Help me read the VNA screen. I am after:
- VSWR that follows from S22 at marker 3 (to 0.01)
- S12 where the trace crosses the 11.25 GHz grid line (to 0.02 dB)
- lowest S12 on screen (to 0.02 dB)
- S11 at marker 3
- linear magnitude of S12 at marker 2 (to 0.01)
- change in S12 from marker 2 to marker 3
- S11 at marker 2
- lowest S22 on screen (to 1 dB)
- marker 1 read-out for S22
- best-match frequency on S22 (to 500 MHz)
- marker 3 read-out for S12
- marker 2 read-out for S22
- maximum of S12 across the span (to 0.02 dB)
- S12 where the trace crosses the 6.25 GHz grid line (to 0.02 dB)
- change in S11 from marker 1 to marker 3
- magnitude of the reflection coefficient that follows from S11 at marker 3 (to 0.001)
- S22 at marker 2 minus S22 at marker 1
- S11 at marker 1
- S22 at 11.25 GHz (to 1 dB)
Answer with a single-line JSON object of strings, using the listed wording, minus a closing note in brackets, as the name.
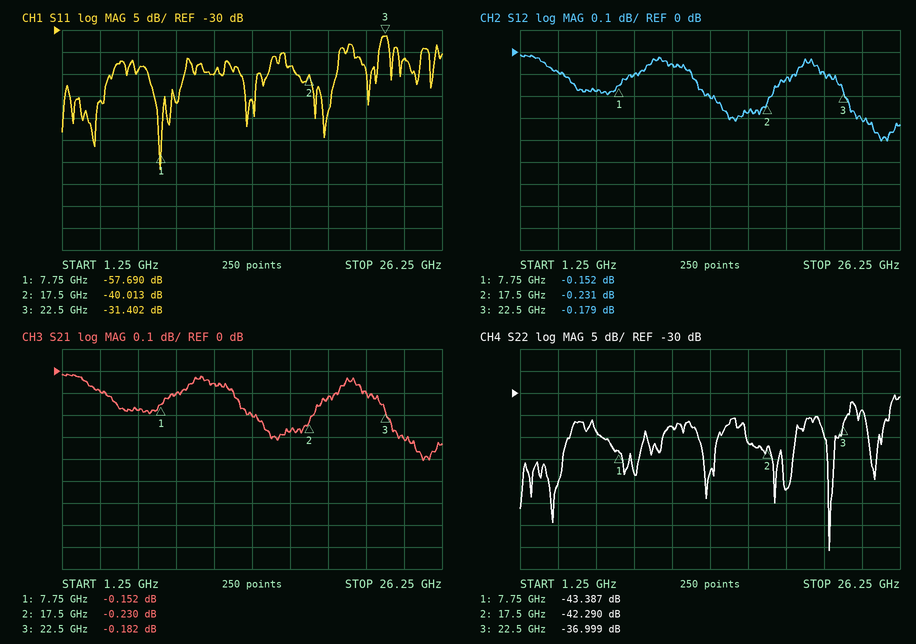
{"VSWR that follows from S22 at marker 3": "1.03", "S12 where the trace crosses the 11.25 GHz grid line": "-0.06 dB", "lowest S12 on screen": "-0.40 dB", "S11 at marker 3": "-31.402 dB", "linear magnitude of S12 at marker 2": "0.97", "change in S12 from marker 2 to marker 3": "0.052 dB", "S11 at marker 2": "-40.013 dB", "lowest S22 on screen": "-66 dB", "marker 1 read-out for S22": "-43.387 dB", "best-match frequency on S22": "21.5 GHz", "marker 3 read-out for S12": "-0.179 dB", "marker 2 read-out for S22": "-42.290 dB", "maximum of S12 across the span": "-0.02 dB", "S12 where the trace crosses the 6.25 GHz grid line": "-0.18 dB", "change in S11 from marker 1 to marker 3": "26.288 dB", "magnitude of the reflection coefficient that follows from S11 at marker 3": "0.027", "S22 at marker 2 minus S22 at marker 1": "1.097 dB", "S11 at marker 1": "-57.690 dB", "S22 at 11.25 GHz": "-38 dB"}
